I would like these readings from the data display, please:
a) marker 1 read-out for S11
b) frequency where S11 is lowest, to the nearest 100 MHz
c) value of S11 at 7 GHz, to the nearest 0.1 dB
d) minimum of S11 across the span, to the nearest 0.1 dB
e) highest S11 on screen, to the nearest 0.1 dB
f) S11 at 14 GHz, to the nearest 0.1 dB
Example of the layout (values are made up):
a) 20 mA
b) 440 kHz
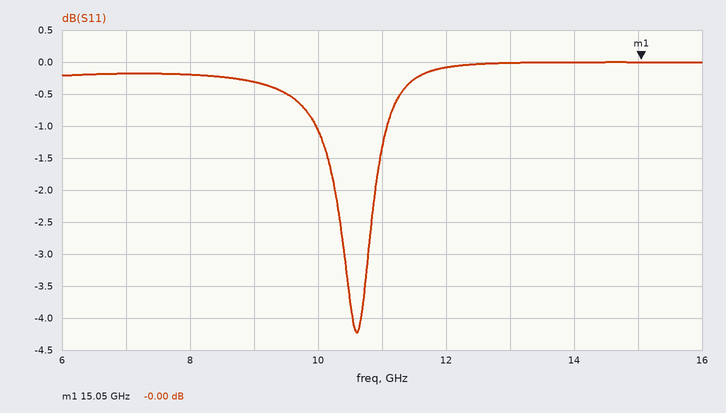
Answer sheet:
a) -0.00 dB
b) 10.6 GHz
c) -0.2 dB
d) -4.2 dB
e) 0.0 dB
f) 0.0 dB
